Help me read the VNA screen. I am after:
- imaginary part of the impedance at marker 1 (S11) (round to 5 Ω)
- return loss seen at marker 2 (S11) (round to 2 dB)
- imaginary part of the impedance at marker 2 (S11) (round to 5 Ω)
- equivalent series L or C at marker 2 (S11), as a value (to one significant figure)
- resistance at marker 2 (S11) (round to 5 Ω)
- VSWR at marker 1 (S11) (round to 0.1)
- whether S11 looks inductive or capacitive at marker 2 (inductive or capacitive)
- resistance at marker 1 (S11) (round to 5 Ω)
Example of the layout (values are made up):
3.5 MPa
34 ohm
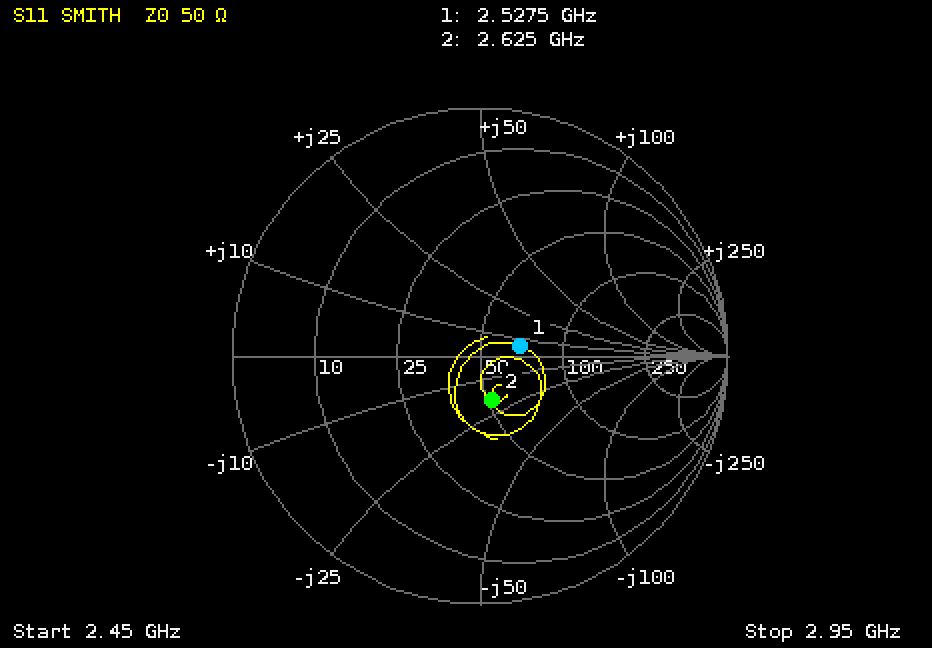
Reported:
+5 Ω
14 dB
-20 Ω
3 pF
50 Ω
1.4
capacitive
70 Ω
